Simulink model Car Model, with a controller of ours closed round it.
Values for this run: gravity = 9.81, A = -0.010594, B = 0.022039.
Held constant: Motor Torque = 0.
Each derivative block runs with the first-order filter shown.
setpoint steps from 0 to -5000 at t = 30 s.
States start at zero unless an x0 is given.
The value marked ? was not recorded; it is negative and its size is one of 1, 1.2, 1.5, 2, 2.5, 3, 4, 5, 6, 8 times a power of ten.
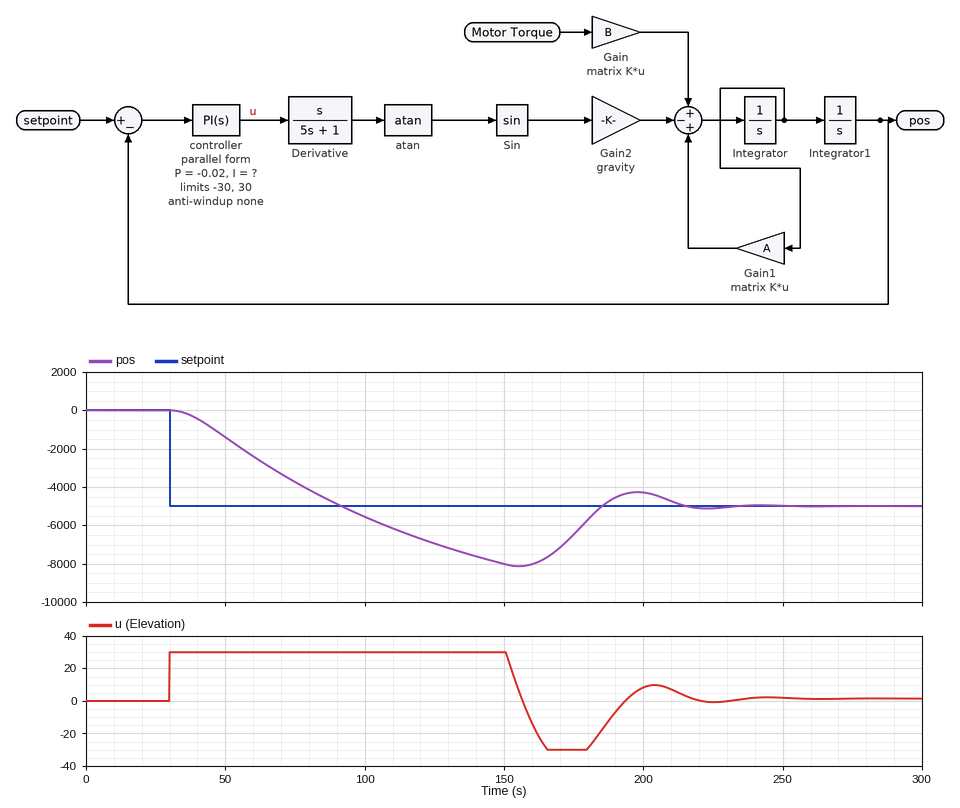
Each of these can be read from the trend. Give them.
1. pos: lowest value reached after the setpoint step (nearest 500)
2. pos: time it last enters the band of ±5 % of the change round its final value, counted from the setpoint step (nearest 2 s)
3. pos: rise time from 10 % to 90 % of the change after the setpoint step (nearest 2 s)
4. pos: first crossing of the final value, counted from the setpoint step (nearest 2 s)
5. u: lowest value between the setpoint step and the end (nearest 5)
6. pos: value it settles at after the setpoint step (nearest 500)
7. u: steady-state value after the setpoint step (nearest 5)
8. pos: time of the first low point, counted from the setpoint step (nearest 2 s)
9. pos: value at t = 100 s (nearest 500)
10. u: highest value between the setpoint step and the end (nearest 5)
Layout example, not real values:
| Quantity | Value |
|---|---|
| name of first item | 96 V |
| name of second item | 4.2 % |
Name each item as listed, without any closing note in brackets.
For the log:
| Quantity | Value |
|---|---|
| pos: lowest value reached after the setpoint step | -8000 |
| pos: time it last enters the band of ±5 % of the change round its final value, counted from the setpoint step | 180 s |
| pos: rise time from 10 % to 90 % of the change after the setpoint step | 44 s |
| pos: first crossing of the final value, counted from the setpoint step | 62 s |
| u: lowest value between the setpoint step and the end | -30 |
| pos: value it settles at after the setpoint step | -5000 |
| u: steady-state value after the setpoint step | 0 |
| pos: time of the first low point, counted from the setpoint step | 126 s |
| pos: value at t = 100 s | -5500 |
| u: highest value between the setpoint step and the end | 30 |
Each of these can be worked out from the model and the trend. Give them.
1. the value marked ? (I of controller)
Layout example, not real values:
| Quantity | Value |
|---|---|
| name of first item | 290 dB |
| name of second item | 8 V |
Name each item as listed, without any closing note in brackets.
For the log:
| Quantity | Value |
|---|---|
| the value marked ? | -0.0015 |
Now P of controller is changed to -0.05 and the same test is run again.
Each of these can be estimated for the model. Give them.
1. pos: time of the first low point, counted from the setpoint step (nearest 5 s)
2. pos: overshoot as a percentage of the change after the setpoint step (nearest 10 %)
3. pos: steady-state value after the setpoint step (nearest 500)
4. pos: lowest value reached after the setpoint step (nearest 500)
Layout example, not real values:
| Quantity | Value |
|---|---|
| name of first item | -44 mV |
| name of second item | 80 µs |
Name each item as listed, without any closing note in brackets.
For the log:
| Quantity | Value |
|---|---|
| pos: time of the first low point, counted from the setpoint step | 110 s |
| pos: overshoot as a percentage of the change after the setpoint step | 50 % |
| pos: steady-state value after the setpoint step | -5000 |
| pos: lowest value reached after the setpoint step | -7500 |
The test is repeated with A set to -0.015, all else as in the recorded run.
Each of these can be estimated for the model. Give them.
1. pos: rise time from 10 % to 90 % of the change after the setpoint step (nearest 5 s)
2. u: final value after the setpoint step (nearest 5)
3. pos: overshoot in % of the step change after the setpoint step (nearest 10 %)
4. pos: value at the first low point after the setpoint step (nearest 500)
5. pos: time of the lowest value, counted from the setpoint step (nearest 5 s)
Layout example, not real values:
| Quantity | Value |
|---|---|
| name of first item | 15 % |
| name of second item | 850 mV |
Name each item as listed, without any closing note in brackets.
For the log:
| Quantity | Value |
|---|---|
| pos: rise time from 10 % to 90 % of the change after the setpoint step | 50 s |
| u: final value after the setpoint step | 15 |
| pos: overshoot in % of the step change after the setpoint step | 50 % |
| pos: value at the first low point after the setpoint step | -7500 |
| pos: time of the lowest value, counted from the setpoint step | 160 s |
